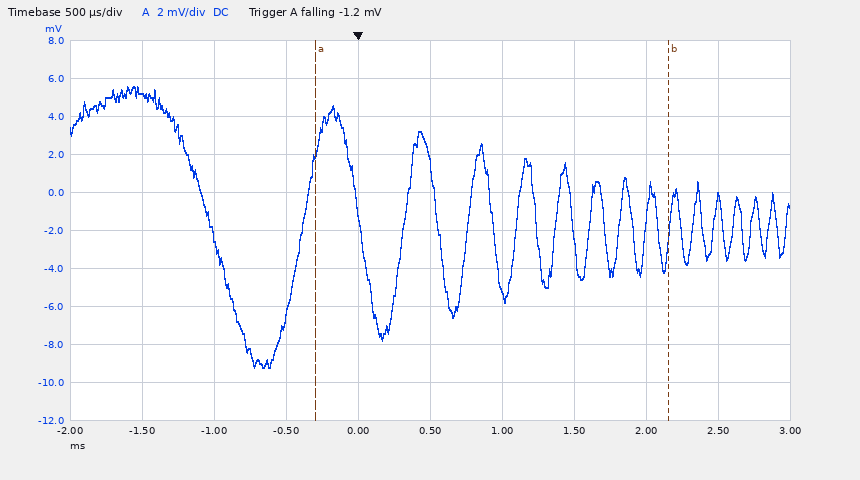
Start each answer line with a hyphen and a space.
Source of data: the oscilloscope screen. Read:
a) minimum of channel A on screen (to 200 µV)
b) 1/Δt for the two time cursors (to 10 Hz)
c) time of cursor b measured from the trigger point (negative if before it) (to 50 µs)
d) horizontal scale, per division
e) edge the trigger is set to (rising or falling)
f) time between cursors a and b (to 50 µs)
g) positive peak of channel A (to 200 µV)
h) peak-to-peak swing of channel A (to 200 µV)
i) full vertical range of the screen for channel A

- -9.2 mV
- 410 Hz
- +2.15 ms
- 500 µs
- falling
- 2.45 ms
- 5.6 mV
- 14.8 mV
- 20 mV
